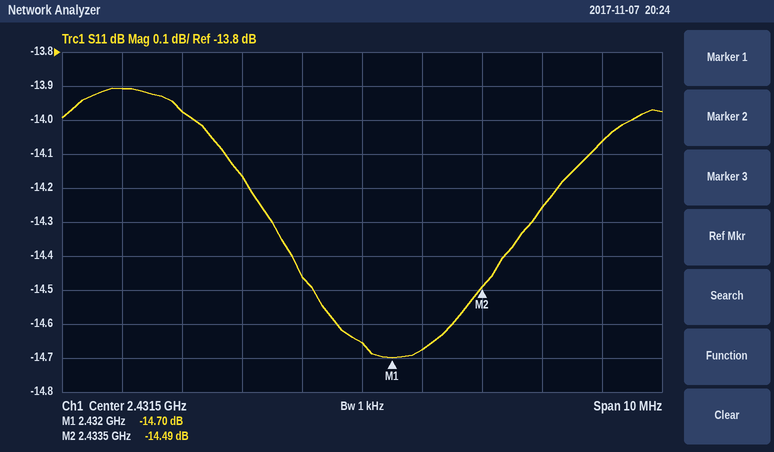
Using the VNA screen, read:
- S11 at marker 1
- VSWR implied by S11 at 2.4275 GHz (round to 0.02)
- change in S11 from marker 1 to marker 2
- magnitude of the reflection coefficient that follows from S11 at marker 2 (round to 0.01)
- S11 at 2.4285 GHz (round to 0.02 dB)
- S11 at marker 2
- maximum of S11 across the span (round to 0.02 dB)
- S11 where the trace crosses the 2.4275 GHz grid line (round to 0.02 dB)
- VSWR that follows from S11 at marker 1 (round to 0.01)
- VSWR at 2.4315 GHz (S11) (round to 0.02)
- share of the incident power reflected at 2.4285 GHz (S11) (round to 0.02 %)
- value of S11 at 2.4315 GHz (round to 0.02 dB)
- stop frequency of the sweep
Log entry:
-14.70 dB
1.50
0.21 dB
0.19
-13.98 dB
-14.49 dB
-13.90 dB
-13.90 dB
1.45
1.46
4.00 %
-14.66 dB
2.4365 GHz
